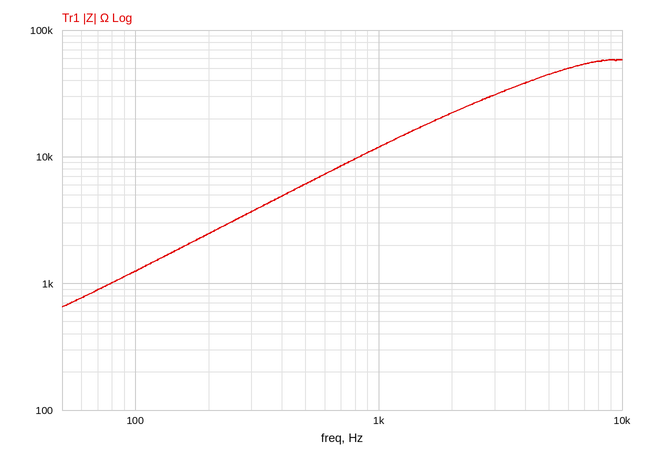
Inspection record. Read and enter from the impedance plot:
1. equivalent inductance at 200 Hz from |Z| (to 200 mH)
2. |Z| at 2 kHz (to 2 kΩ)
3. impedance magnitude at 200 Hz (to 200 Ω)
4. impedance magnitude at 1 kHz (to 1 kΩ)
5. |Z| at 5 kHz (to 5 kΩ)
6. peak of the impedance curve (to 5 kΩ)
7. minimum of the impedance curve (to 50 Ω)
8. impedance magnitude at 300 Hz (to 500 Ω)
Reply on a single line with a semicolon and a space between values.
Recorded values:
2.0 H; 22 kΩ; 2.4 kΩ; 12 kΩ; 45 kΩ; 60 kΩ; 650 Ω; 3.5 kΩ
